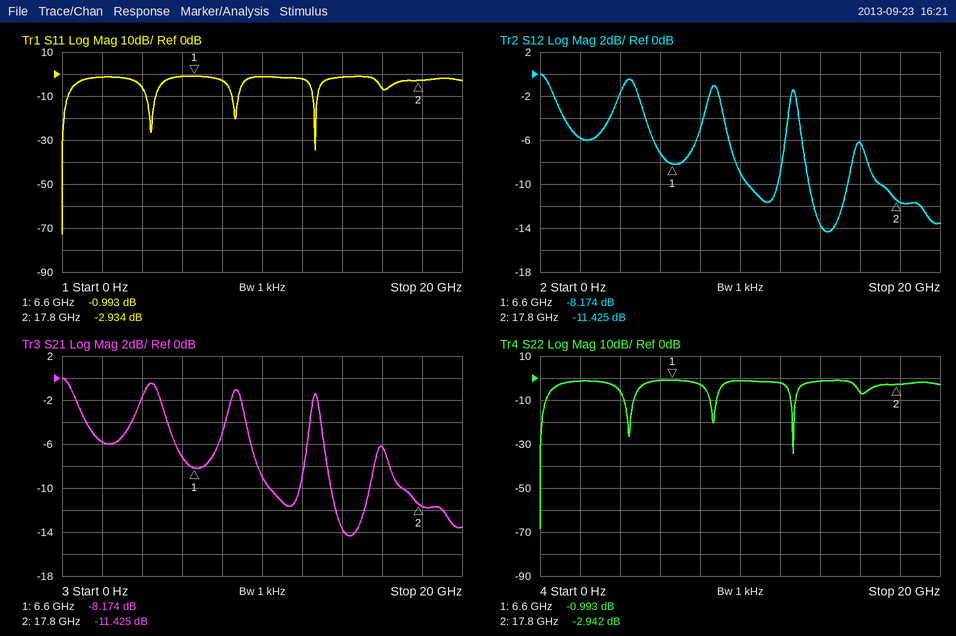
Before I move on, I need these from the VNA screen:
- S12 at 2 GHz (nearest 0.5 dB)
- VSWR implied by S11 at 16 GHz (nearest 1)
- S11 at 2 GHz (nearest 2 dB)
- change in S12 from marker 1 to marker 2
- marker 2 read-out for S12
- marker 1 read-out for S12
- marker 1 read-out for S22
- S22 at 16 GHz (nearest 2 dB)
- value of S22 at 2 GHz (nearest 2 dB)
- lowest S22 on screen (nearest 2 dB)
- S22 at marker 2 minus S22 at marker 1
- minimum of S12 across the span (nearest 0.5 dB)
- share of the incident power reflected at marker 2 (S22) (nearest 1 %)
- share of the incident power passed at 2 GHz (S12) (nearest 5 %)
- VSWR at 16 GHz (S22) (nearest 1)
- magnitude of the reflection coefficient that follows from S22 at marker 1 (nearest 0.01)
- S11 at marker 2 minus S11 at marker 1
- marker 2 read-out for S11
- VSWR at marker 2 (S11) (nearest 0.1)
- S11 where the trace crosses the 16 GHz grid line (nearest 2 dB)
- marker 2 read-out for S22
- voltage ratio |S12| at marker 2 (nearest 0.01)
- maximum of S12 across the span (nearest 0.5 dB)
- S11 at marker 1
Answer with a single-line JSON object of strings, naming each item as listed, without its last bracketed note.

{"S12 at 2 GHz": "-6.0 dB", "VSWR implied by S11 at 16 GHz": "3", "S11 at 2 GHz": "-2 dB", "change in S12 from marker 1 to marker 2": "-3.251 dB", "marker 2 read-out for S12": "-11.425 dB", "marker 1 read-out for S12": "-8.174 dB", "marker 1 read-out for S22": "-0.993 dB", "S22 at 16 GHz": "-6 dB", "value of S22 at 2 GHz": "-2 dB", "lowest S22 on screen": "-68 dB", "S22 at marker 2 minus S22 at marker 1": "-1.949 dB", "minimum of S12 across the span": "-14.5 dB", "share of the incident power reflected at marker 2 (S22)": "51 %", "share of the incident power passed at 2 GHz (S12)": "25 %", "VSWR at 16 GHz (S22)": "3", "magnitude of the reflection coefficient that follows from S22 at marker 1": "0.89", "S11 at marker 2 minus S11 at marker 1": "-1.941 dB", "marker 2 read-out for S11": "-2.934 dB", "VSWR at marker 2 (S11)": "6.0", "S11 where the trace crosses the 16 GHz grid line": "-6 dB", "marker 2 read-out for S22": "-2.942 dB", "voltage ratio |S12| at marker 2": "0.27", "maximum of S12 across the span": "0.0 dB", "S11 at marker 1": "-0.993 dB"}
